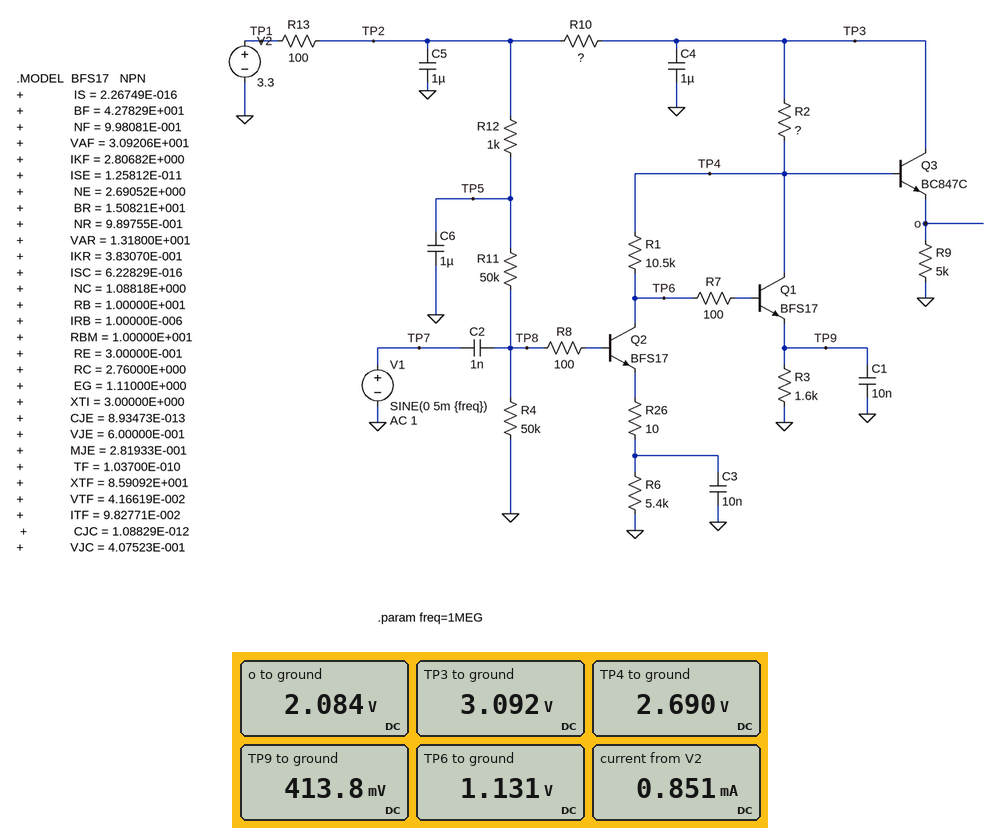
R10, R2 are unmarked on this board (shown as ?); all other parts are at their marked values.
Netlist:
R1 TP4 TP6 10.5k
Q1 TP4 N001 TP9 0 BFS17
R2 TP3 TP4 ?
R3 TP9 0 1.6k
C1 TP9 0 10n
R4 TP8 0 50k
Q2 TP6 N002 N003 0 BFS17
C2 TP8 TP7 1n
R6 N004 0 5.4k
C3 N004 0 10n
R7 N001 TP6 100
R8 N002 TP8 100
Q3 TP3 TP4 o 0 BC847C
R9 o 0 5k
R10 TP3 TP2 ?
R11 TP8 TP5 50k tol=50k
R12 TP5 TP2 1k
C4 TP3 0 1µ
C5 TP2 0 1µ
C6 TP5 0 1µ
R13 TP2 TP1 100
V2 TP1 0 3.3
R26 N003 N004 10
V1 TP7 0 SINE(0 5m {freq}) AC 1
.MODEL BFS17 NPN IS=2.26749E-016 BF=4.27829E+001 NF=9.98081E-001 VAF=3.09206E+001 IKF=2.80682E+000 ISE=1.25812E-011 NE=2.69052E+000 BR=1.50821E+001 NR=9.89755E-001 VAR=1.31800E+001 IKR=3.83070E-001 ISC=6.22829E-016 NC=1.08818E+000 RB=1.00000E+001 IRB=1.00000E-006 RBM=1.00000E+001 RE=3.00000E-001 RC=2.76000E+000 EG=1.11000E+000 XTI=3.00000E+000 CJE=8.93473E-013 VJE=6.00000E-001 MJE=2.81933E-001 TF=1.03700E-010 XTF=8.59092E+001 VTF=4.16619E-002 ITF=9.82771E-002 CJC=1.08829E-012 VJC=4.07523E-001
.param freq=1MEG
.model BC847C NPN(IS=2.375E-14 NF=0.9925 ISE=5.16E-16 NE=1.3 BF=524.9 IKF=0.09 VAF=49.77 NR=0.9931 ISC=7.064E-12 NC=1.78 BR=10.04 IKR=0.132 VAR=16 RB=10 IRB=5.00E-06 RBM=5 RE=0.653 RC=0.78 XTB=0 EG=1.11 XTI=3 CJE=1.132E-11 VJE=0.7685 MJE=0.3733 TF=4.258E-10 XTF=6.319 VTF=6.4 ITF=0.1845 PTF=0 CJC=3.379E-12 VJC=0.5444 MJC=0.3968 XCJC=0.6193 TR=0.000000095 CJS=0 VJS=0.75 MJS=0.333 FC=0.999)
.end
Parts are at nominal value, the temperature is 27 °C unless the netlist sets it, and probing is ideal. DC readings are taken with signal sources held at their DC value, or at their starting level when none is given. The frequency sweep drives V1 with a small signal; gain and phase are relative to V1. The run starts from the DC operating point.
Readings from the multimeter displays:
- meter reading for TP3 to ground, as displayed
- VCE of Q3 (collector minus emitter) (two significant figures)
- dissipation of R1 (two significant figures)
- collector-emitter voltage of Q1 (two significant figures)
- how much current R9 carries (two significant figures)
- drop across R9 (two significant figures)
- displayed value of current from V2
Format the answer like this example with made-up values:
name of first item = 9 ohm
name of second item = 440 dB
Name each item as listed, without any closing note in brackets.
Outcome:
meter reading for TP3 to ground, as displayed = 3.092 V
VCE of Q3 (collector minus emitter) = 1.0 V
dissipation of R1 = 230 µW
collector-emitter voltage of Q1 = 2.3 V
how much current R9 carries = 420 µA
drop across R9 = 2.1 V
displayed value of current from V2 = 0.851 mA
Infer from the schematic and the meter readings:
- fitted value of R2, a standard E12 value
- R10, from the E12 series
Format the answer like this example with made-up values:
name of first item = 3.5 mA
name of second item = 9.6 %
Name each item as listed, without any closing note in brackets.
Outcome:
fitted value of R2, a standard E12 value = 1 kΩ
R10, from the E12 series = 150 Ω
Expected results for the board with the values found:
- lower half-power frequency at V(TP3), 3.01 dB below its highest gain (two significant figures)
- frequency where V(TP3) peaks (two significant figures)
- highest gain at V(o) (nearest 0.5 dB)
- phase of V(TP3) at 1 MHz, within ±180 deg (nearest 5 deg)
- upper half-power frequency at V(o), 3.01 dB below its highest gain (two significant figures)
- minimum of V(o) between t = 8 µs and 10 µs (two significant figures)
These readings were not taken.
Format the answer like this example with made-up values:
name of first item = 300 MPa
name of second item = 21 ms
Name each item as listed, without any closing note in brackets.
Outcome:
lower half-power frequency at V(TP3), 3.01 dB below its highest gain = 14 kHz
frequency where V(TP3) peaks = 47 kHz
highest gain at V(o) = 31.5 dB
phase of V(TP3) at 1 MHz, within ±180 deg = -85 deg
upper half-power frequency at V(o), 3.01 dB below its highest gain = 17 MHz
minimum of V(o) between t = 8 µs and 10 µs = 1.9 V
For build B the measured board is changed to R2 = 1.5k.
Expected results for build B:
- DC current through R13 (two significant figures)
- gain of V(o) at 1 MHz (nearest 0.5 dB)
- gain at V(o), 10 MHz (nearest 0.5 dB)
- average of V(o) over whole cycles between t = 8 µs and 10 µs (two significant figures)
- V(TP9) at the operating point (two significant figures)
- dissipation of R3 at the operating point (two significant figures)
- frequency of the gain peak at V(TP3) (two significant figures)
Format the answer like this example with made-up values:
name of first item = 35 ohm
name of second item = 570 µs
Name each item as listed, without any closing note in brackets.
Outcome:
DC current through R13 = 780 µA
gain of V(o) at 1 MHz = 32.0 dB
gain at V(o), 10 MHz = 31.0 dB
average of V(o) over whole cycles between t = 8 µs and 10 µs = 2.0 V
V(TP9) at the operating point = 330 mV
dissipation of R3 at the operating point = 67 µW
frequency of the gain peak at V(TP3) = 43 kHz
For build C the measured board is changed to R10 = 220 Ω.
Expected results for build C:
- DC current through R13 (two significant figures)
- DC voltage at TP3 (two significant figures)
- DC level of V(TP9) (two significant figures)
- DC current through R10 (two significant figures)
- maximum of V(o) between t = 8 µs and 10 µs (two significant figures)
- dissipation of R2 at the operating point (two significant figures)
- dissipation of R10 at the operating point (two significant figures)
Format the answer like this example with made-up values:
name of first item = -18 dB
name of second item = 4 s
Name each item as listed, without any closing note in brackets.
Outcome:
DC current through R13 = 830 µA
DC voltage at TP3 = 3.0 V
DC level of V(TP9) = 390 mV
DC current through R10 = 790 µA
maximum of V(o) between t = 8 µs and 10 µs = 2.2 V
dissipation of R2 at the operating point = 150 µW
dissipation of R10 at the operating point = 140 µW
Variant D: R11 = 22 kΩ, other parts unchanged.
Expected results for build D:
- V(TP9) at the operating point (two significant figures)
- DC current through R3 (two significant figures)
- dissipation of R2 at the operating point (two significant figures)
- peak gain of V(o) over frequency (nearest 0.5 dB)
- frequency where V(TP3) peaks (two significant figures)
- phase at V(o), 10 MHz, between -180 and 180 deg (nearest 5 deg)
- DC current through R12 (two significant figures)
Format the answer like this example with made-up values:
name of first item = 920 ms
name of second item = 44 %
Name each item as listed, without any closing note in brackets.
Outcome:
V(TP9) at the operating point = 330 mV
DC current through R3 = 210 µA
dissipation of R2 at the operating point = 130 µW
peak gain of V(o) over frequency = 15.0 dB
frequency where V(TP3) peaks = 190 kHz
phase at V(o), 10 MHz, between -180 and 180 deg = -70 deg
DC current through R12 = 65 µA
